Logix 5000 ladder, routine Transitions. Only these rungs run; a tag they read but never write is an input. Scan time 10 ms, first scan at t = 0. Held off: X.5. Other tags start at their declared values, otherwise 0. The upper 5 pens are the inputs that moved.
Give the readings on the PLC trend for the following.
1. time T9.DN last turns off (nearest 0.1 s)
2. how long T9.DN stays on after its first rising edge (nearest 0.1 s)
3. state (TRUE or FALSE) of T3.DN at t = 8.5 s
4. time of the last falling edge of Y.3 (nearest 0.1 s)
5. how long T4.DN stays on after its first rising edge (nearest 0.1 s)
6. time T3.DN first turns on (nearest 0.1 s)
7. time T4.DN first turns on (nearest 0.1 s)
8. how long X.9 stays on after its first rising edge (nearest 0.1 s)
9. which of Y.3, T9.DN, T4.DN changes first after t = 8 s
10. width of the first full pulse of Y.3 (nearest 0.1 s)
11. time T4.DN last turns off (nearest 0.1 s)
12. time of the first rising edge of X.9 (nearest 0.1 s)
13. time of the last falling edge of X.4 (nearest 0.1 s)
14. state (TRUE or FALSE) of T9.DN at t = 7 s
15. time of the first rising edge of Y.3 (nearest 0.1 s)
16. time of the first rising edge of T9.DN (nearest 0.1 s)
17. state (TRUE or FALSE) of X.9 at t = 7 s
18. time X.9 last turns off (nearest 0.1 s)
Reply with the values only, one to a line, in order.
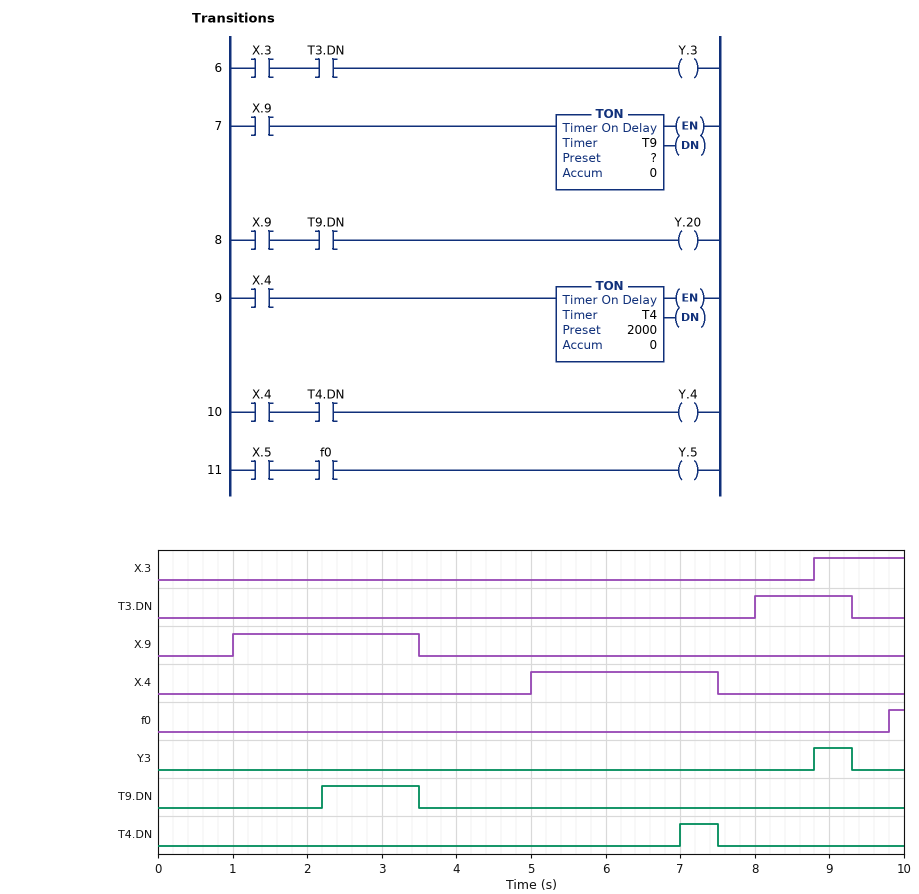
3.5 s
1.3 s
TRUE
9.3 s
0.5 s
8.0 s
7.0 s
2.5 s
Y.3
0.5 s
7.5 s
1.0 s
7.5 s
FALSE
8.8 s
2.2 s
FALSE
3.5 s
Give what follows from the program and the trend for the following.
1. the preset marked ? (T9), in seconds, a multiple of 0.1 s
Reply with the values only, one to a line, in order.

1.2 s
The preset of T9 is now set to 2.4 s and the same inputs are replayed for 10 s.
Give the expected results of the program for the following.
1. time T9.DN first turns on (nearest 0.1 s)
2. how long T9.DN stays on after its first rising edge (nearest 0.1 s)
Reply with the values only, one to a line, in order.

3.4 s
0.1 s
